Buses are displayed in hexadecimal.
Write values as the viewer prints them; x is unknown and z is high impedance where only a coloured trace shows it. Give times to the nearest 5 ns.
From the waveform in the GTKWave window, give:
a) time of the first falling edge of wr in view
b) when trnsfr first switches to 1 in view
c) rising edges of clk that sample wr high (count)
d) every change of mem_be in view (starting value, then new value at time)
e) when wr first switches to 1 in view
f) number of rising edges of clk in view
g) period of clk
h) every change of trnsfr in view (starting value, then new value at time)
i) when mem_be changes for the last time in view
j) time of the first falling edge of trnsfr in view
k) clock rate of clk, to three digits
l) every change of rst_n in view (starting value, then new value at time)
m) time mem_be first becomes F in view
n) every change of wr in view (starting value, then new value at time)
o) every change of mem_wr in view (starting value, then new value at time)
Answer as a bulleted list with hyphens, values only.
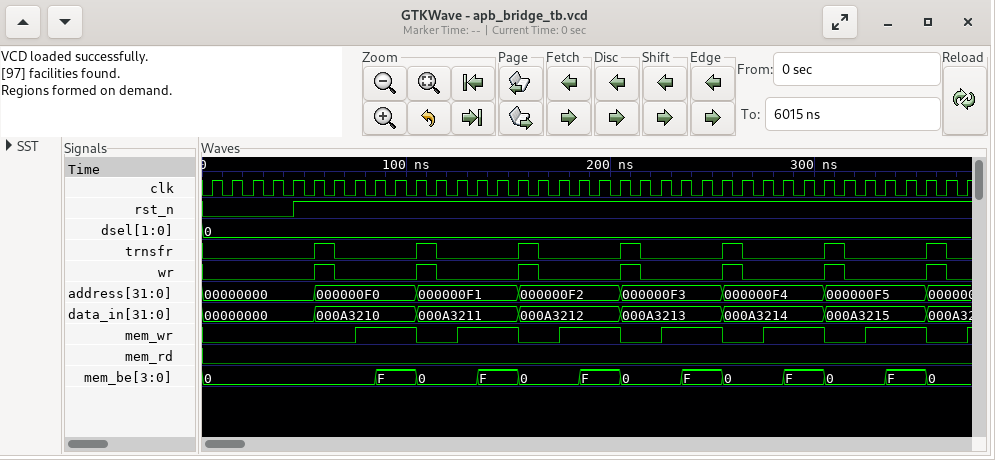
- 65 ns
- 55 ns
- 7
- 0, F at 85 ns, 0 at 105 ns, F at 135 ns, 0 at 155 ns, F at 185 ns, 0 at 205 ns, F at 235 ns, 0 at 255 ns, F at 285 ns, 0 at 305 ns, F at 335 ns, 0 at 355 ns
- 55 ns
- 38
- 10 ns
- 0, 1 at 55 ns, 0 at 65 ns, 1 at 105 ns, 0 at 115 ns, 1 at 155 ns, 0 at 165 ns, 1 at 205 ns, 0 at 215 ns, 1 at 255 ns, 0 at 265 ns, 1 at 305 ns, 0 at 315 ns, 1 at 355 ns, 0 at 365 ns
- 355 ns
- 65 ns
- 100 MHz
- 0, 1 at 45 ns
- 85 ns
- 0, 1 at 55 ns, 0 at 65 ns, 1 at 105 ns, 0 at 115 ns, 1 at 155 ns, 0 at 165 ns, 1 at 205 ns, 0 at 215 ns, 1 at 255 ns, 0 at 265 ns, 1 at 305 ns, 0 at 315 ns, 1 at 355 ns, 0 at 365 ns
- 0, 1 at 75 ns, 0 at 105 ns, 1 at 125 ns, 0 at 155 ns, 1 at 175 ns, 0 at 205 ns, 1 at 225 ns, 0 at 255 ns, 1 at 275 ns, 0 at 305 ns, 1 at 325 ns, 0 at 355 ns, 1 at 375 ns
